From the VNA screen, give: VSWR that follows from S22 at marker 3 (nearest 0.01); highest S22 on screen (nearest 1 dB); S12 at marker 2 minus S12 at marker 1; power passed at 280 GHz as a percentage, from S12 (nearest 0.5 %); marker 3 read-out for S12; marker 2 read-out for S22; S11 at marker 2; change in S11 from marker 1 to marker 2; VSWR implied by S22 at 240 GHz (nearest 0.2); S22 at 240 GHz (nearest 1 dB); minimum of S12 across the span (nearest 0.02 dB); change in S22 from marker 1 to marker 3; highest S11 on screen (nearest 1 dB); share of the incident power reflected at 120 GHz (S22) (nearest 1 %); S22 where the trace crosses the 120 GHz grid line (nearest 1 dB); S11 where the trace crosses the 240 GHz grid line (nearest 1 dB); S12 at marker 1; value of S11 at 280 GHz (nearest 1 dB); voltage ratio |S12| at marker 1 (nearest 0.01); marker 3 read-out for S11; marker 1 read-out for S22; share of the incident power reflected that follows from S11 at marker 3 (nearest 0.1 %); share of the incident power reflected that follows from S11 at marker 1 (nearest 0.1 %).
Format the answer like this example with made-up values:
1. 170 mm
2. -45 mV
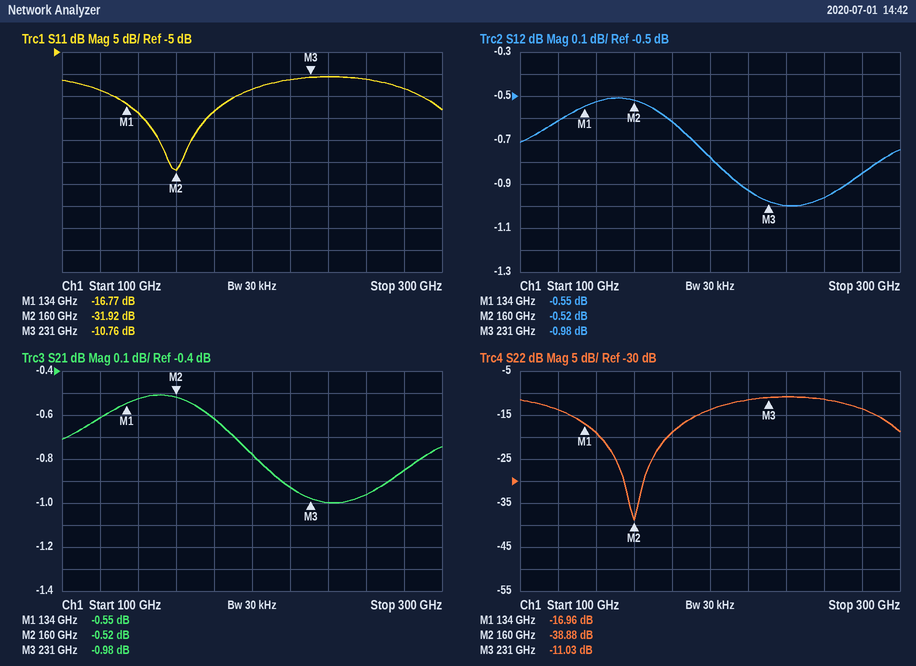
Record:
1. 1.78
2. -11 dB
3. 0.03 dB
4. 82.0 %
5. -0.98 dB
6. -38.88 dB
7. -31.92 dB
8. -15.15 dB
9. 1.8
10. -11 dB
11. -1.00 dB
12. 5.93 dB
13. -11 dB
14. 4 %
15. -14 dB
16. -11 dB
17. -0.55 dB
18. -13 dB
19. 0.94
20. -10.76 dB
21. -16.96 dB
22. 8.4 %
23. 2.1 %
